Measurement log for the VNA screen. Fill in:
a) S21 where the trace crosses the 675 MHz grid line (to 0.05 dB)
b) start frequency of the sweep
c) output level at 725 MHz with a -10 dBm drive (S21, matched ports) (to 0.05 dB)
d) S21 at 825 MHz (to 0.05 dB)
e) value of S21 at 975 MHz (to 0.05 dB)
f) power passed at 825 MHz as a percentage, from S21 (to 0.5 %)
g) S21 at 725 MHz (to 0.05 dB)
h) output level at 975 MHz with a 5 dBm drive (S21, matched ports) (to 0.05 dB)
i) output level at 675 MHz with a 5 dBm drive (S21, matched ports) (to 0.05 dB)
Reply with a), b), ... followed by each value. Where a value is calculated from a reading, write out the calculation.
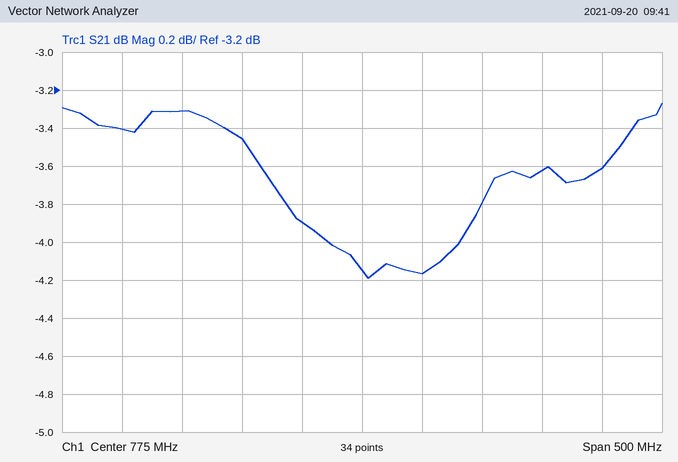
a) -3.45 dB
b) 525 MHz
c) -10 dBm + (-3.90 dB) = -13.90 dBm
d) -4.15 dB
e) -3.60 dB
f) 10^(-4.15/10) ≈ 38.5 %
g) -3.90 dB
h) 5 dBm + (-3.60 dB) = 1.40 dBm
i) 5 dBm + (-3.45 dB) = 1.55 dBm
